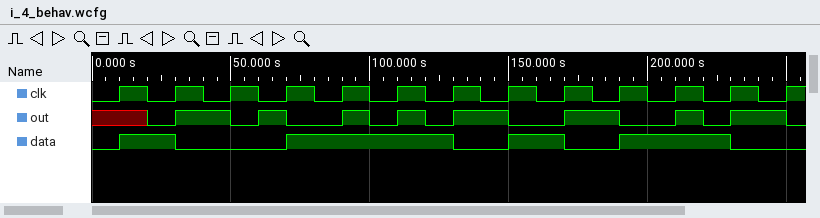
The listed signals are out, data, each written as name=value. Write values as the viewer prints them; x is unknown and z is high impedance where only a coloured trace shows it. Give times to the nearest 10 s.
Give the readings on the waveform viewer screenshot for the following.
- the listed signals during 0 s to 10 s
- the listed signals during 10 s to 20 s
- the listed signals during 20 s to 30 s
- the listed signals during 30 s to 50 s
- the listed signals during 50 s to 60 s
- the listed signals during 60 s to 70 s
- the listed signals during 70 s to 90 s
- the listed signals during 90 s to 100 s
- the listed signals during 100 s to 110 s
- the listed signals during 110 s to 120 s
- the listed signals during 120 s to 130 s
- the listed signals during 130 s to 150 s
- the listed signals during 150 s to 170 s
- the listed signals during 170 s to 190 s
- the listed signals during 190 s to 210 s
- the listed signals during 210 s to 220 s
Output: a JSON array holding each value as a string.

["out=x, data=0", "out=x, data=1", "out=0, data=1", "out=1, data=0", "out=0, data=0", "out=1, data=0", "out=0, data=1", "out=1, data=1", "out=0, data=1", "out=1, data=1", "out=0, data=1", "out=1, data=0", "out=0, data=1", "out=1, data=0", "out=0, data=1", "out=1, data=1"]
